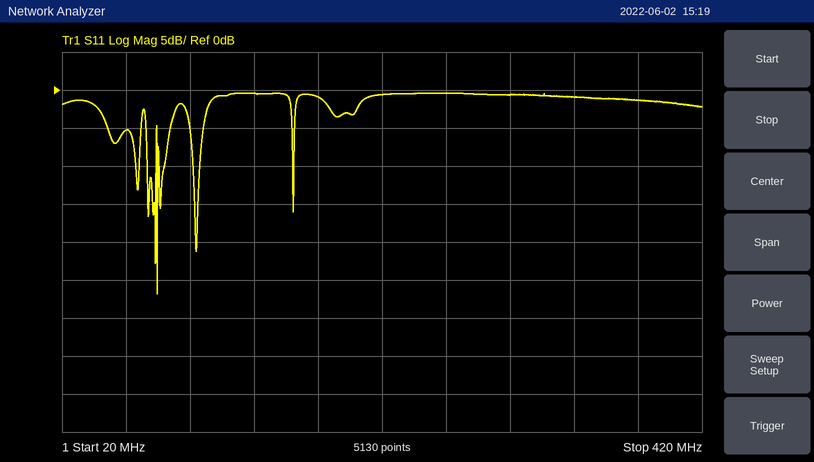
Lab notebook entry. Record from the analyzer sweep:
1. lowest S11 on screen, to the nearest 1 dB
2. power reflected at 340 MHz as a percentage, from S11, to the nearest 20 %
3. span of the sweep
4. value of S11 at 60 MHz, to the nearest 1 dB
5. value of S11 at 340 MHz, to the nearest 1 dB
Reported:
-27 dB
80 %
400 MHz
-5 dB
-1 dB
